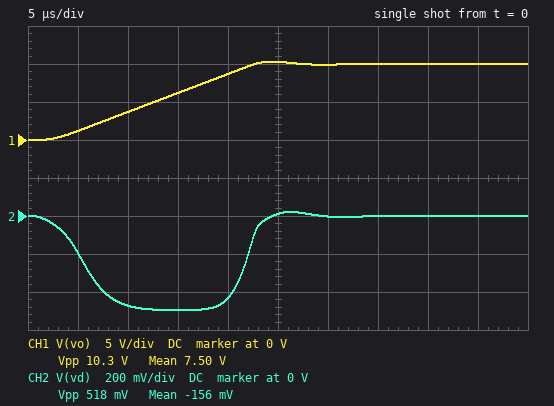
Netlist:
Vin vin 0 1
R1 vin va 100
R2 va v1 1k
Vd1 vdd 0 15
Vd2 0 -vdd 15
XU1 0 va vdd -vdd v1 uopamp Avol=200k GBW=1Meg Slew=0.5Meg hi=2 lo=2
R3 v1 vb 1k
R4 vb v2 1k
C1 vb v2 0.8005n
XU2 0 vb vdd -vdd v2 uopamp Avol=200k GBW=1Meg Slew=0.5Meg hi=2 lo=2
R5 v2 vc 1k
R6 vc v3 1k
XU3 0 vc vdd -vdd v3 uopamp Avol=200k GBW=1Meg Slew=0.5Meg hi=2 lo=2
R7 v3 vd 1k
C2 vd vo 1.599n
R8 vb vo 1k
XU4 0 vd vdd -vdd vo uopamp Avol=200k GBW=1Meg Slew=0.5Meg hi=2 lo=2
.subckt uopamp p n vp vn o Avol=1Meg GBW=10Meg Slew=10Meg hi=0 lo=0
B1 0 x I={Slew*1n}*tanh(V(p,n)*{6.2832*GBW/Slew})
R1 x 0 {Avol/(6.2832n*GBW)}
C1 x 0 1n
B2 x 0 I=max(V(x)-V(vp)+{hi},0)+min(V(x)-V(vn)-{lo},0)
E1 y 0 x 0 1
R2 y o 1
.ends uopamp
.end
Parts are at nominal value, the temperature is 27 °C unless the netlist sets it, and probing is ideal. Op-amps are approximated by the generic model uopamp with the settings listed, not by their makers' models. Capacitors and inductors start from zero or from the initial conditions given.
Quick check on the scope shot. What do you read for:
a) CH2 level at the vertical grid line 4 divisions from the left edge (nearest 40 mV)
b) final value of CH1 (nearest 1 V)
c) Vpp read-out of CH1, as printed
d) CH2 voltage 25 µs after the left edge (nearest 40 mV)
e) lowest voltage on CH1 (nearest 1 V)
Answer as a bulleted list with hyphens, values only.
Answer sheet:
- -440 mV
- 10 V
- 10.3 V
- 0 V
- 0 V
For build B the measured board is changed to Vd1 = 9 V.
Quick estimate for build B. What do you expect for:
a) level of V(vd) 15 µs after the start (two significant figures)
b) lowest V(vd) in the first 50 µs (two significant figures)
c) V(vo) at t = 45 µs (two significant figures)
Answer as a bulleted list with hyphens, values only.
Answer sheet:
- -500 mV
- -3.0 V
- 7.0 V
